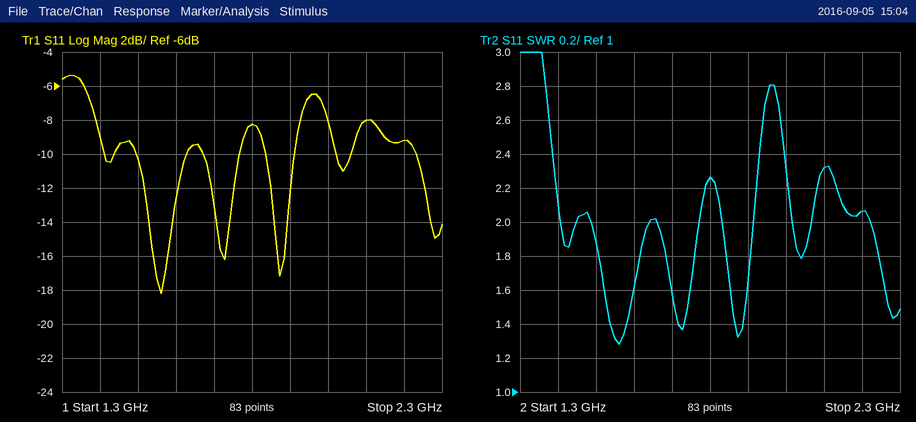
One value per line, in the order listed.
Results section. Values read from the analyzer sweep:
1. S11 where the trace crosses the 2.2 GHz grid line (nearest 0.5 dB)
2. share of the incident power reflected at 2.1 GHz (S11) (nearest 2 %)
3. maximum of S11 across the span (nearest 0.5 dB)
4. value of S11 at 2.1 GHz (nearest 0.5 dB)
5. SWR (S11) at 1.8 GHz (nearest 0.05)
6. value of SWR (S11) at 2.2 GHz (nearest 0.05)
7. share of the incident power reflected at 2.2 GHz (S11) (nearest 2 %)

-9.0 dB
16 %
-5.5 dB
-8.0 dB
2.25
2.05
12 %
